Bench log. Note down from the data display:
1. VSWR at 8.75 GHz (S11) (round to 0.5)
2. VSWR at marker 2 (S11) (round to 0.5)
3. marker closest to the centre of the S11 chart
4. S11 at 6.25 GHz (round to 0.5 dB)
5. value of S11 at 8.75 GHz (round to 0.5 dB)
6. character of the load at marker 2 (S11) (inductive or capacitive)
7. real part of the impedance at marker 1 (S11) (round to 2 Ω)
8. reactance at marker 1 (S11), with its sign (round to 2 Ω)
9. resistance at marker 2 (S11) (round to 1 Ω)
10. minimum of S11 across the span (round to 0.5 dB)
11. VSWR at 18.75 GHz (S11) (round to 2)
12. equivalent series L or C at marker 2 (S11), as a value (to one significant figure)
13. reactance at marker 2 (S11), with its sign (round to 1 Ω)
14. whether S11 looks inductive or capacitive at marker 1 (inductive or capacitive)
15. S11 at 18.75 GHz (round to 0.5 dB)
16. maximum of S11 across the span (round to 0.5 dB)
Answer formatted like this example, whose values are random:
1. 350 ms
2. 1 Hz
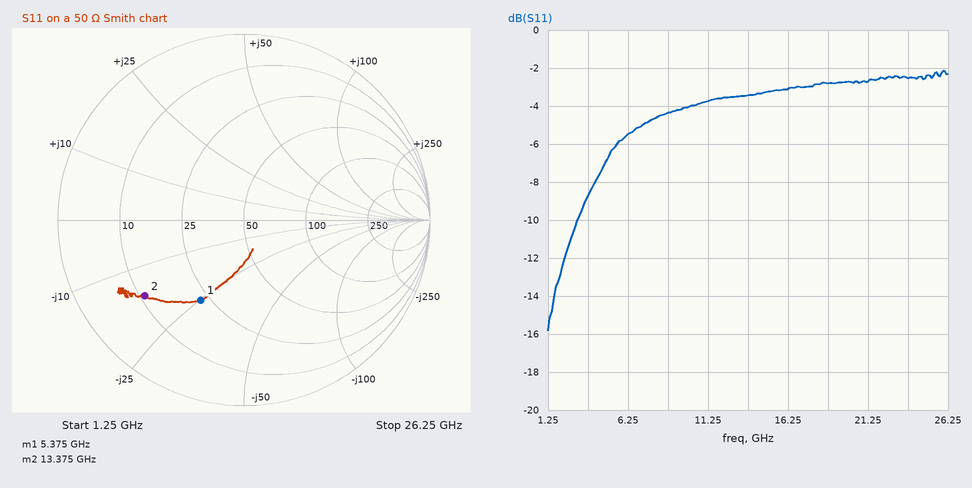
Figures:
1. 4.0
2. 5.0
3. marker 1
4. -5.5 dB
5. -4.5 dB
6. capacitive
7. 22 Ω
8. -26 Ω
9. 11 Ω
10. -16.0 dB
11. 6
12. 700 fF
13. -16 Ω
14. capacitive
15. -3.0 dB
16. -2.0 dB
